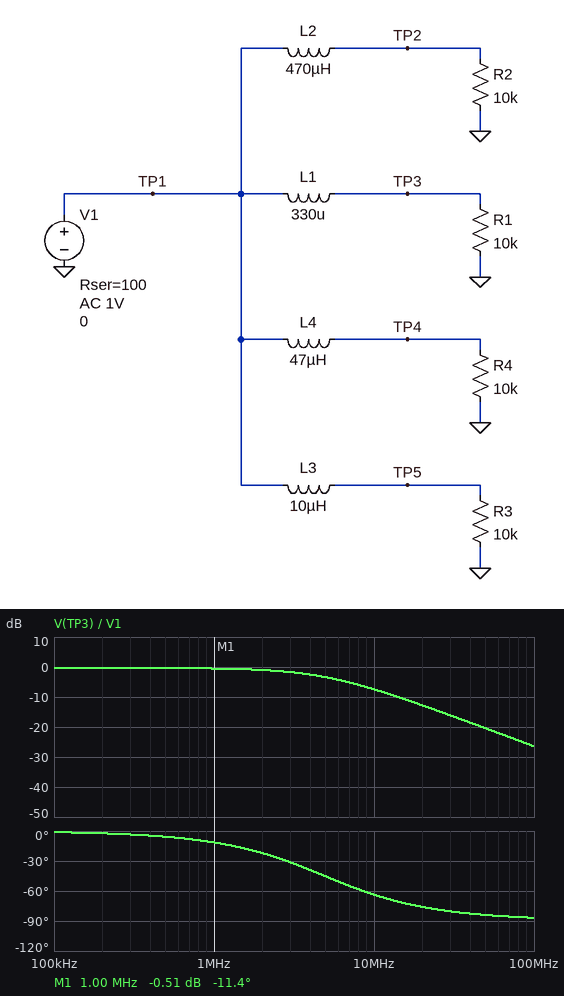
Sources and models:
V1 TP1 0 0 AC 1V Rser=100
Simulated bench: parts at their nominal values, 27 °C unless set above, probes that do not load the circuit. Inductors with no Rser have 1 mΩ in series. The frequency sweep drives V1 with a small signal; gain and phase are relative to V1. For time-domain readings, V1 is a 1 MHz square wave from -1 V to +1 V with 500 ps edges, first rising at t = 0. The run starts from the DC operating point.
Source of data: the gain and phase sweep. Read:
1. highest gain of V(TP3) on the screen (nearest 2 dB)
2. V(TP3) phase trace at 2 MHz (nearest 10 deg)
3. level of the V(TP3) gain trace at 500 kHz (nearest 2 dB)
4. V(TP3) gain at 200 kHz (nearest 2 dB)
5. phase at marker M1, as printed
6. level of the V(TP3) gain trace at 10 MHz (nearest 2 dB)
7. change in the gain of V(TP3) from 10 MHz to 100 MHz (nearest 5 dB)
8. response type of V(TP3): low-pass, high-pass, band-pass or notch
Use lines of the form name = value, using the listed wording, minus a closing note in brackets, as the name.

highest gain of V(TP3) on the screen = 0 dB
V(TP3) phase trace at 2 MHz = -20 deg
level of the V(TP3) gain trace at 500 kHz = 0 dB
V(TP3) gain at 200 kHz = 0 dB
phase at marker M1, as printed = -11.4 deg
level of the V(TP3) gain trace at 10 MHz = -8 dB
change in the gain of V(TP3) from 10 MHz to 100 MHz = -20 dB
response type of V(TP3): low-pass, high-pass, band-pass or notch = low-pass
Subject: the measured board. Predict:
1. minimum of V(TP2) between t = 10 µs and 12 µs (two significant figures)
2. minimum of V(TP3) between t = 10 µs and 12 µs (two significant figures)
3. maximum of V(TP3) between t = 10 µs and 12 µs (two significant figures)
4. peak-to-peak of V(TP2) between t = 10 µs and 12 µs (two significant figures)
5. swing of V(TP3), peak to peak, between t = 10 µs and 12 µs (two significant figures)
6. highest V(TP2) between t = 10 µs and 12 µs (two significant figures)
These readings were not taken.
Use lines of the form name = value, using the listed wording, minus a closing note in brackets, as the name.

minimum of V(TP2) between t = 10 µs and 12 µs = -960 mV
minimum of V(TP3) between t = 10 µs and 12 µs = -960 mV
maximum of V(TP3) between t = 10 µs and 12 µs = 960 mV
peak-to-peak of V(TP2) between t = 10 µs and 12 µs = 1.9 V
swing of V(TP3), peak to peak, between t = 10 µs and 12 µs = 1.9 V
highest V(TP2) between t = 10 µs and 12 µs = 960 mV
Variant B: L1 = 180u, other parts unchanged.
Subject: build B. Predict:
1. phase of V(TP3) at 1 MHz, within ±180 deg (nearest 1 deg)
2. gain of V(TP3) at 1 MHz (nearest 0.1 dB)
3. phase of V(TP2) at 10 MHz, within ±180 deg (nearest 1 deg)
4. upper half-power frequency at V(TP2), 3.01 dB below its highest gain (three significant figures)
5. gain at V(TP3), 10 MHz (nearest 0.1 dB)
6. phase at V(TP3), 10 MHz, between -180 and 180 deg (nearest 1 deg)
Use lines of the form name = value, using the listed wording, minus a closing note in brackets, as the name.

phase of V(TP3) at 1 MHz, within ±180 deg = -6 deg
gain of V(TP3) at 1 MHz = -0.4 dB
phase of V(TP2) at 10 MHz, within ±180 deg = -71 deg
upper half-power frequency at V(TP2), 3.01 dB below its highest gain = 3.43 MHz
gain at V(TP3), 10 MHz = -3.8 dB
phase at V(TP3), 10 MHz, between -180 and 180 deg = -48 deg
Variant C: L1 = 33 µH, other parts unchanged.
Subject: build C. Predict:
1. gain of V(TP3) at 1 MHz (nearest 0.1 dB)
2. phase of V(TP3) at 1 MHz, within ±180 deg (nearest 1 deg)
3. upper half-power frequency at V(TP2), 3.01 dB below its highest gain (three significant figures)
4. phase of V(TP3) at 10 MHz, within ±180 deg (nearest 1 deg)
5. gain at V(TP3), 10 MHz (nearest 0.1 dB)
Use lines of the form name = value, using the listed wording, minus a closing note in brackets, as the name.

gain of V(TP3) at 1 MHz = -0.3 dB
phase of V(TP3) at 1 MHz, within ±180 deg = -1 deg
upper half-power frequency at V(TP2), 3.01 dB below its highest gain = 3.42 MHz
phase of V(TP3) at 10 MHz, within ±180 deg = -11 deg
gain at V(TP3), 10 MHz = -0.4 dB
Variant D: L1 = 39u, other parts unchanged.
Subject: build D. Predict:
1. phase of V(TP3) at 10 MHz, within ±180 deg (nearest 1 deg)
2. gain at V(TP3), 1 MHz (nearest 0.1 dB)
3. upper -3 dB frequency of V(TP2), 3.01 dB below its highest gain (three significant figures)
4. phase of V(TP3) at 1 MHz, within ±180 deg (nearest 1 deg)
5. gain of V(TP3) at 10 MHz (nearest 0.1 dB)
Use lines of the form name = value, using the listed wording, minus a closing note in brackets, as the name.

phase of V(TP3) at 10 MHz, within ±180 deg = -13 deg
gain at V(TP3), 1 MHz = -0.3 dB
upper -3 dB frequency of V(TP2), 3.01 dB below its highest gain = 3.42 MHz
phase of V(TP3) at 1 MHz, within ±180 deg = -1 deg
gain of V(TP3) at 10 MHz = -0.5 dB
